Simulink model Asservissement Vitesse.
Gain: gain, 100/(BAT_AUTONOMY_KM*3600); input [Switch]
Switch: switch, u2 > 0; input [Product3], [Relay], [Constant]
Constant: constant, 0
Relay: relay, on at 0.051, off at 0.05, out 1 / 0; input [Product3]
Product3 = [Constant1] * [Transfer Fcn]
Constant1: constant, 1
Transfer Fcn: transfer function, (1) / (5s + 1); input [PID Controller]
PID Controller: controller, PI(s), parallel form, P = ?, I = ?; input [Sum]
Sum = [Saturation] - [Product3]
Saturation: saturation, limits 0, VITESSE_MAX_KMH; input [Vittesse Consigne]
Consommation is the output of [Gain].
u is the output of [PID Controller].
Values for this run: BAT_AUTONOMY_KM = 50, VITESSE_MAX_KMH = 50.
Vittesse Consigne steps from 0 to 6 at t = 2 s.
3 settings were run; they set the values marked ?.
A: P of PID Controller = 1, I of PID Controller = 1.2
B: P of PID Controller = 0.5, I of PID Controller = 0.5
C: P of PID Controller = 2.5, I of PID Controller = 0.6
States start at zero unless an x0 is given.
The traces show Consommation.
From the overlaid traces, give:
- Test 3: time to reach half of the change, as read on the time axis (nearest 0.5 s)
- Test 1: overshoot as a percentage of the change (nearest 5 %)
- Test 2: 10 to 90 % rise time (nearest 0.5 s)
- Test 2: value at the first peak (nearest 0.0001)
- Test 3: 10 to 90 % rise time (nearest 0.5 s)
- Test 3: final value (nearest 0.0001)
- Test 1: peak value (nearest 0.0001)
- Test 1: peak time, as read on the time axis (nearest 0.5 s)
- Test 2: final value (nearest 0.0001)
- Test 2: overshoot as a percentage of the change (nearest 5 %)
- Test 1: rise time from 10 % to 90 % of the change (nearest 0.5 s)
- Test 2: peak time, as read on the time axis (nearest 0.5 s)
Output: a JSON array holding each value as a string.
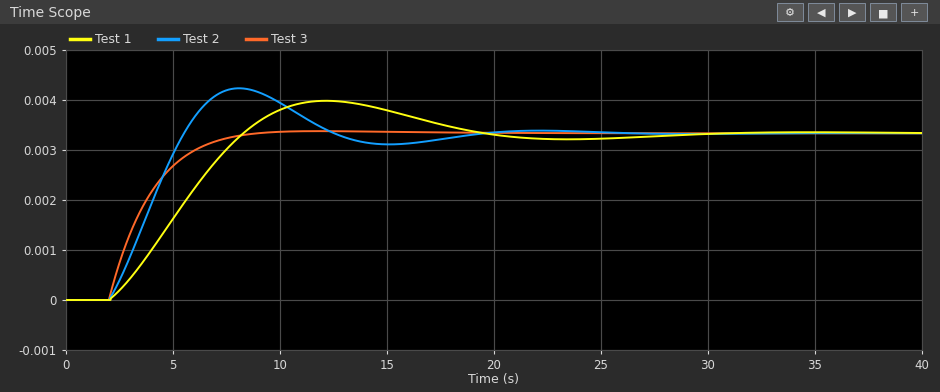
["3.5 s", "20 %", "2.5 s", "0.0042", "4.0 s", "0.0033", "0.0040", "12.0 s", "0.0033", "25 %", "4.5 s", "8.0 s"]
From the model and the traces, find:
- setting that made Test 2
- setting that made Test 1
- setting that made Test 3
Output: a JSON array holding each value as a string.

["A", "B", "C"]
